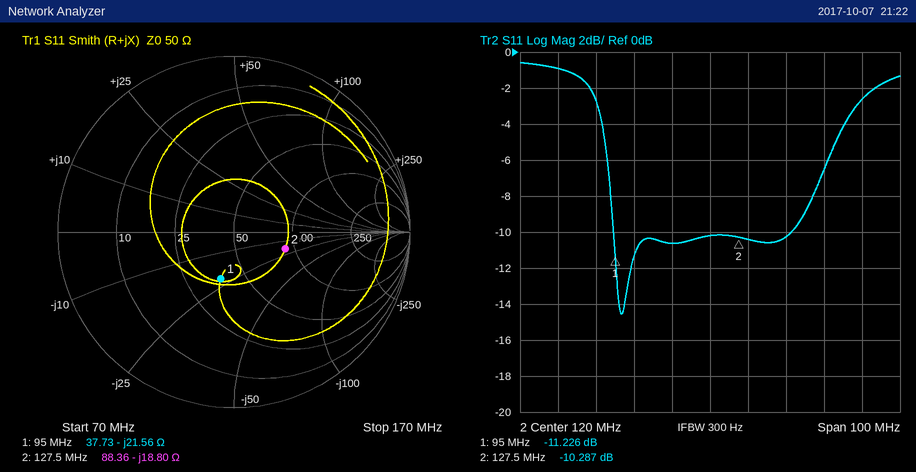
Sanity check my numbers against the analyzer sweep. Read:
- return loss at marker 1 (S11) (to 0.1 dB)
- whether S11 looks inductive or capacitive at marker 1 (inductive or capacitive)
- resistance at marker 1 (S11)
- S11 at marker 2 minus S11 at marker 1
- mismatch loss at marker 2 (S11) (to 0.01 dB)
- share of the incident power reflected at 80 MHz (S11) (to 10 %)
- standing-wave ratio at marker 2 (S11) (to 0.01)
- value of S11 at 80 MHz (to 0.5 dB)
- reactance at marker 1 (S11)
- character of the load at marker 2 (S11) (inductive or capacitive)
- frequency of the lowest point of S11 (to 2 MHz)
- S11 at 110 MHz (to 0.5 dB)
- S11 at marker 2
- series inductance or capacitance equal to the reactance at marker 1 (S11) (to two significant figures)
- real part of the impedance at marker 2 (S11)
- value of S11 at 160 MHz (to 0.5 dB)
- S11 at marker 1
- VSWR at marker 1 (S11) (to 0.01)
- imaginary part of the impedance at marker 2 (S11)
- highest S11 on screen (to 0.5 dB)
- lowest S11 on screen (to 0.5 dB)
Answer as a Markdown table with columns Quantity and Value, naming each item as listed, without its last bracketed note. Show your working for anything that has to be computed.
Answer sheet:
| Quantity | Value |
|---|---|
| return loss at marker 1 (S11) | 11.2 dB |
| whether S11 looks inductive or capacitive at marker 1 | capacitive |
| resistance at marker 1 | 37.73 Ω |
| S11 at marker 2 minus S11 at marker 1 | -10.287 − (-11.226) = 0.939 dB |
| mismatch loss at marker 2 (S11) | −10 log10(1 − 10^(-10.287/10)) ≈ 0.43 dB |
| share of the incident power reflected at 80 MHz (S11) | 10^(-1/10) ≈ 79.4 %, so 80 % to the nearest 10 % |
| standing-wave ratio at marker 2 (S11) | 1.88 |
| value of S11 at 80 MHz | -1.0 dB |
| reactance at marker 1 | -21.56 Ω |
| character of the load at marker 2 (S11) | capacitive |
| frequency of the lowest point of S11 | 96 MHz |
| S11 at 110 MHz | -10.5 dB |
| S11 at marker 2 | -10.287 dB |
| series inductance or capacitance equal to the reactance at marker 1 (S11) | C = 1/(2π × 95 MHz × 21.56 Ω) ≈ 78 pF |
| real part of the impedance at marker 2 | 88.36 Ω |
| value of S11 at 160 MHz | -2.5 dB |
| S11 at marker 1 | -11.226 dB |
| VSWR at marker 1 (S11) | (1 + 0.2746)/(1 − 0.2746) ≈ 1.76 |
| imaginary part of the impedance at marker 2 | -18.80 Ω |
| highest S11 on screen | -0.5 dB |
| lowest S11 on screen | -14.5 dB |
